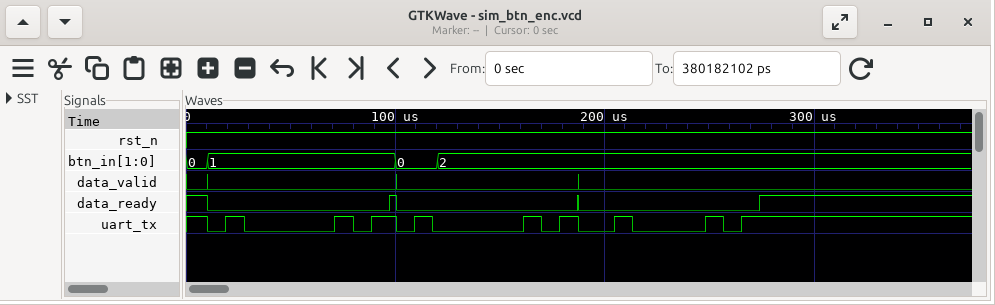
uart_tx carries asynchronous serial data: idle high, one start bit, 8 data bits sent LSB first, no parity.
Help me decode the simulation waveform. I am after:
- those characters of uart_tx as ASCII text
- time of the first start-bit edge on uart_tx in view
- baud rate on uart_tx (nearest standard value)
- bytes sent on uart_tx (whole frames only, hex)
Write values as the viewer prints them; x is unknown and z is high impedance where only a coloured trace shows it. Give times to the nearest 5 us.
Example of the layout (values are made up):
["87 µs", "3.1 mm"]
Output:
["\"AAB\"", "10 us", "115200 baud", "41, 41, 42"]
